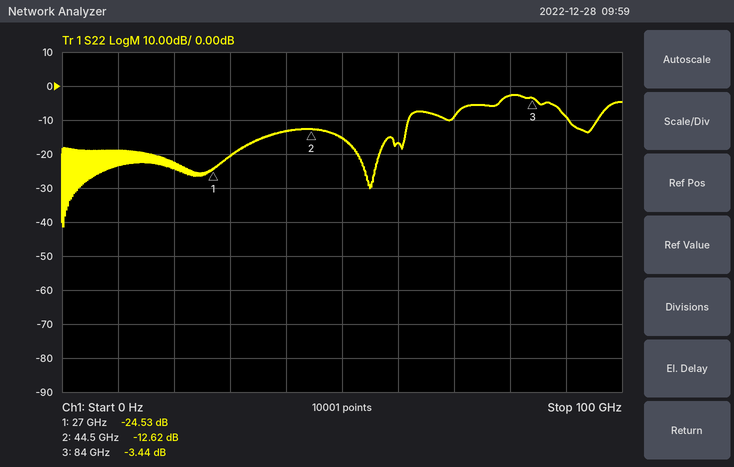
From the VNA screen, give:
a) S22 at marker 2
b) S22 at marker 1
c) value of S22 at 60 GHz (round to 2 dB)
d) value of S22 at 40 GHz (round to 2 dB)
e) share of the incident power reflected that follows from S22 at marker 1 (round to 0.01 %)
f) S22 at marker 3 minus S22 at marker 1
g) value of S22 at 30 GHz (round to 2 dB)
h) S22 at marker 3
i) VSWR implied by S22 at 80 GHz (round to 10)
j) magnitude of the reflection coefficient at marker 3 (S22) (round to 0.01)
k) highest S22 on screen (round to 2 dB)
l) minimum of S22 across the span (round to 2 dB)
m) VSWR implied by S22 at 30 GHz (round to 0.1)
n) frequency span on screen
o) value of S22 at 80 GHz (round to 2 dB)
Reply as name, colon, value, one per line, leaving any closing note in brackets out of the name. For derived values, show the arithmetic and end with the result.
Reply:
S22 at marker 2: -12.62 dB
S22 at marker 1: -24.53 dB
value of S22 at 60 GHz: -16 dB
value of S22 at 40 GHz: -14 dB
share of the incident power reflected that follows from S22 at marker 1: 10^(-24.53/10) ≈ 0.35 %
S22 at marker 3 minus S22 at marker 1: -3.44 − (-24.53) = 21.09 dB
value of S22 at 30 GHz: -20 dB
S22 at marker 3: -3.44 dB
VSWR implied by S22 at 80 GHz: |Γ| = 10^(-2/20) = 0.7943; VSWR = (1 + 0.7943)/(1 − 0.7943) ≈ 8.72, so 10 to the nearest 10
magnitude of the reflection coefficient at marker 3 (S22): 10^(-3.44/20) ≈ 0.67
highest S22 on screen: -2 dB
minimum of S22 across the span: -42 dB
VSWR implied by S22 at 30 GHz: |Γ| = 10^(-20/20) = 0.1000; VSWR = (1 + 0.1000)/(1 − 0.1000) ≈ 1.2
frequency span on screen: 100 GHz
value of S22 at 80 GHz: -2 dB
